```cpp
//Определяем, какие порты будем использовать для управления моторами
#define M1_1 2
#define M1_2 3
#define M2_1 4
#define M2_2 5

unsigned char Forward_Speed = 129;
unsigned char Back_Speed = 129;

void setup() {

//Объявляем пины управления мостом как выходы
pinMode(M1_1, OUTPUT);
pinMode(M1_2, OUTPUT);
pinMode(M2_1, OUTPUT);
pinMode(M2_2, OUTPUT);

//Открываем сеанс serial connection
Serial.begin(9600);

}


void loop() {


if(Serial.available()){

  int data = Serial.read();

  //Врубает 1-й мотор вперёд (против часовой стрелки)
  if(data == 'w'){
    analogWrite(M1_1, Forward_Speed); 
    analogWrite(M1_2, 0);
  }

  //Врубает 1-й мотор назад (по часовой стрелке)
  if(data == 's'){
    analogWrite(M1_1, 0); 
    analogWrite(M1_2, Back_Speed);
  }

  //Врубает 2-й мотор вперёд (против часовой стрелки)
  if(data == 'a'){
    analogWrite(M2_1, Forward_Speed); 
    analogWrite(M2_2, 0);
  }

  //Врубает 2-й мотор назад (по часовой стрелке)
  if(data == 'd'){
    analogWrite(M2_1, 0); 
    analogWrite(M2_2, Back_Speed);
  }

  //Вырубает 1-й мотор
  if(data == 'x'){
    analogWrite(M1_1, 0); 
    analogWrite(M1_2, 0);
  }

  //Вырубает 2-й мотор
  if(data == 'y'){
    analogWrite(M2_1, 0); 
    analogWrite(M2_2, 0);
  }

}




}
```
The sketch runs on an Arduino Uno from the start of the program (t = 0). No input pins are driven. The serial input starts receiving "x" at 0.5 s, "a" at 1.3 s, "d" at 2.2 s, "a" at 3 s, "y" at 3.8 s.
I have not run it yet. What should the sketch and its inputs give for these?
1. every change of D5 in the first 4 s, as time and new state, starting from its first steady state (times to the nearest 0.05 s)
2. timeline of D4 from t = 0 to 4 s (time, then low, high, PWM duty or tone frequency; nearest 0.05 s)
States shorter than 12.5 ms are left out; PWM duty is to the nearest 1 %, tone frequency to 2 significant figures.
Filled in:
0 s low; 2.2 s PWM 51 %; 3 s low
0 s low; 1.3 s high; 2.2 s low; 3 s high; 3.8 s low
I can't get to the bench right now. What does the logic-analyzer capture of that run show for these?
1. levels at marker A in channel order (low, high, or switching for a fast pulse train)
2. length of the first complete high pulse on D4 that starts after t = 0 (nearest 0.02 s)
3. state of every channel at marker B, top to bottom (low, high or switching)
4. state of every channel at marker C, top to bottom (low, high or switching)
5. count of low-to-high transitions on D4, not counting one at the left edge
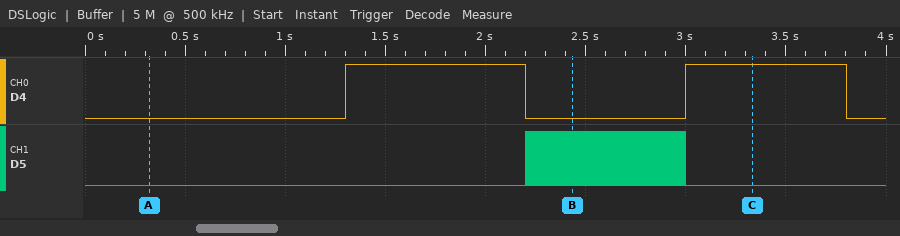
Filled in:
D4 low, D5 low
0.90 s
D4 low, D5 switching
D4 high, D5 low
2
